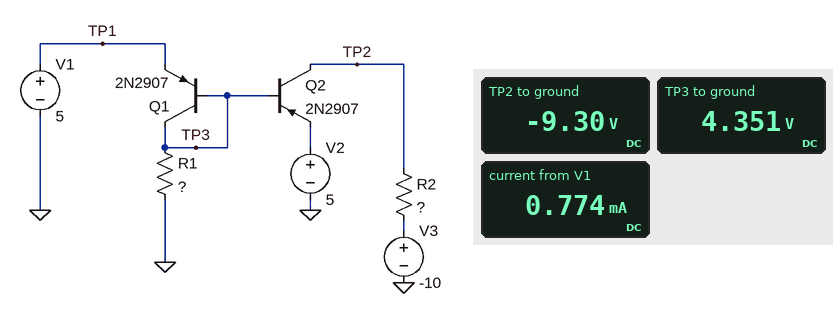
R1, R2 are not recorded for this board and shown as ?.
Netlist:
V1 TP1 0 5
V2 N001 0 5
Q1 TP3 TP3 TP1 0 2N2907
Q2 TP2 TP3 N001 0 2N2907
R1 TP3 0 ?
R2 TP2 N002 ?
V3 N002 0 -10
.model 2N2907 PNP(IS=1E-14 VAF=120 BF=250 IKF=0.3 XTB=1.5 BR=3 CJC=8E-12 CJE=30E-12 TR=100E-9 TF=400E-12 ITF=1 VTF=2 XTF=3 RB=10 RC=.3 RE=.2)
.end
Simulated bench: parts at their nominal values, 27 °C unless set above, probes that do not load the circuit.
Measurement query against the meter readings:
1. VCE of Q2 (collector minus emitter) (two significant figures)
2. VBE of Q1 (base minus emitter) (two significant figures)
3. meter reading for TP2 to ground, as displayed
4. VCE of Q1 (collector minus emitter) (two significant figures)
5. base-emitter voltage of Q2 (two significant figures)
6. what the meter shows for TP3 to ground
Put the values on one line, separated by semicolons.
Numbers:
-14 V; -650 mV; -9.30 V; -650 mV; -650 mV; 4.351 V
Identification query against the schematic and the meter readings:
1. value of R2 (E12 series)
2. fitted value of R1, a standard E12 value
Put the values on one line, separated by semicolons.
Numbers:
820 Ω; 5.6 kΩ
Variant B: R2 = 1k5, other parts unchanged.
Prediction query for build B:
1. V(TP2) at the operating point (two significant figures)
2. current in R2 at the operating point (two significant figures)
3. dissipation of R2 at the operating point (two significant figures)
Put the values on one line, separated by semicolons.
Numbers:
-8.7 V; 850 µA; 1.1 mW
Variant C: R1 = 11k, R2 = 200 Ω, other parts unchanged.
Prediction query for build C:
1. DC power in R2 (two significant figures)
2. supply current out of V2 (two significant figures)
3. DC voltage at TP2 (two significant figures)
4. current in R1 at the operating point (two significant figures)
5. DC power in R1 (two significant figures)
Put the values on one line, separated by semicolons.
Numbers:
39 µW; 440 µA; -9.9 V; 400 µA; 1.7 mW
